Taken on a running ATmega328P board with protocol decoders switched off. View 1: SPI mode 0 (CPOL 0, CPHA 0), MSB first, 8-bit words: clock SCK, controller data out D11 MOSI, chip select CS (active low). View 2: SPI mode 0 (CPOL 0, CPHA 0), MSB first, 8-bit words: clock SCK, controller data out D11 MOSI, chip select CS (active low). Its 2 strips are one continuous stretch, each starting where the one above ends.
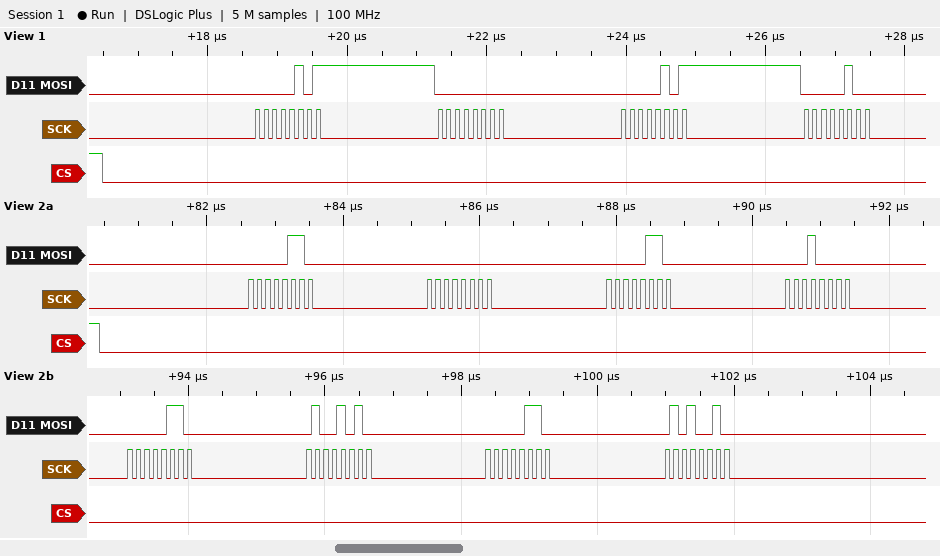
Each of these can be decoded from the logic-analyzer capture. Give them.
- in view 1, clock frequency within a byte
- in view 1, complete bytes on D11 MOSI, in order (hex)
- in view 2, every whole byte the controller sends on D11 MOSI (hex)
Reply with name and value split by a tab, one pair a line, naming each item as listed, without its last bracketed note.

in view 1, clock frequency within a byte	8 MHz
in view 1, complete bytes on D11 MOSI, in order	05 00 05 04
in view 2, every whole byte the controller sends on D11 MOSI	0x06 0x00 0x06 0x10 0x06 0x4A 0x06 0x52
